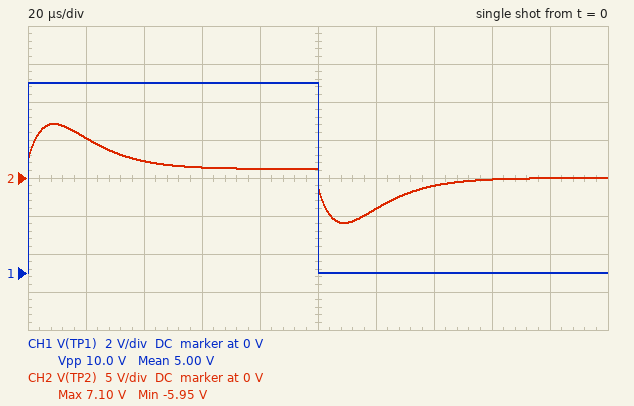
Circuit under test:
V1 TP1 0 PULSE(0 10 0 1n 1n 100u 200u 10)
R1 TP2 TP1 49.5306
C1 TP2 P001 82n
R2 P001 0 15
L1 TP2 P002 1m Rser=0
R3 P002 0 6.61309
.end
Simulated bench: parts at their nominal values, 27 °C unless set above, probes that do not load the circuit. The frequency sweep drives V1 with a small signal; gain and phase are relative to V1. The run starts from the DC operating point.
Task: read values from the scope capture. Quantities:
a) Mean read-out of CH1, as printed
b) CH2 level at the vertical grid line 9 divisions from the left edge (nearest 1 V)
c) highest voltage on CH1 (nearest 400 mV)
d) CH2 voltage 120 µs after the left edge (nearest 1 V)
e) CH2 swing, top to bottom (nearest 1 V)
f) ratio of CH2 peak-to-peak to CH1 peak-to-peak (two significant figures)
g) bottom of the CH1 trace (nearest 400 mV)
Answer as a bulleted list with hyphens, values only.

- 5.00 V
- 0 V
- 10.0 V
- -4 V
- 13 V
- 1.3
- 0 V
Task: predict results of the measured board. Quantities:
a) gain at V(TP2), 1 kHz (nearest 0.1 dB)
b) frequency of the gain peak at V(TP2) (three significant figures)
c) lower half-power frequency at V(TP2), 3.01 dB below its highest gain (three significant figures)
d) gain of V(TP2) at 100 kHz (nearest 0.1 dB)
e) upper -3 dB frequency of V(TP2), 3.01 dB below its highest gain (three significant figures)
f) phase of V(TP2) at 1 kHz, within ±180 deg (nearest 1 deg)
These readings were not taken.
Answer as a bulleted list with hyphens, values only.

- -15.8 dB
- 16.6 kHz
- 6.73 kHz
- -8.6 dB
- 42.0 kHz
- 37 deg
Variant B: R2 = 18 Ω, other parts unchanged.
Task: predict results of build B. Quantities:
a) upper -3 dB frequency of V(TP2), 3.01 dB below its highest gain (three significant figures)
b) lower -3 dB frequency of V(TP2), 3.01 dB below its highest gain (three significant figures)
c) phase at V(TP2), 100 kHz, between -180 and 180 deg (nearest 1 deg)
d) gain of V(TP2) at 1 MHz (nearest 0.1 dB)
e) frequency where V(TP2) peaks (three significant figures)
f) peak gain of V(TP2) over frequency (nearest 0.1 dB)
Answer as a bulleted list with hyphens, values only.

- 41.7 kHz
- 6.65 kHz
- -30 deg
- -11.4 dB
- 16.3 kHz
- -0.8 dB
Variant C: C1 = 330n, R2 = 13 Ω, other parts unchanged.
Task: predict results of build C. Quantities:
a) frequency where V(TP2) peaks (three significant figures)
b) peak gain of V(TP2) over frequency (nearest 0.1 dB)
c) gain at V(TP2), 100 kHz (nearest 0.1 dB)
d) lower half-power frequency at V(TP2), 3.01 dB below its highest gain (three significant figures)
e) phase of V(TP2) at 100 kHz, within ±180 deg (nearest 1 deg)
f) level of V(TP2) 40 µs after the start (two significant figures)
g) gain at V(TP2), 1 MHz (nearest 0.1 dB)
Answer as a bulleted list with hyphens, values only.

- 8.41 kHz
- -2.3 dB
- -13.1 dB
- 4.59 kHz
- -15 deg
- 3.8 V
- -13.6 dB
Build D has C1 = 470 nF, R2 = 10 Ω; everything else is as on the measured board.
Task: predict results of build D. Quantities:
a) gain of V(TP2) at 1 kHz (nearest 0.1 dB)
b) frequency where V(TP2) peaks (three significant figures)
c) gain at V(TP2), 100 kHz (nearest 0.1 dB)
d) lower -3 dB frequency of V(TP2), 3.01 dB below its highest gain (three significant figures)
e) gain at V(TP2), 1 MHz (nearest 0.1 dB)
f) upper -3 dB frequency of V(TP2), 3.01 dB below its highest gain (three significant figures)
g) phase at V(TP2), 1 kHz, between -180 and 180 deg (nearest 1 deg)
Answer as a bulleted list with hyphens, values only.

- -15.7 dB
- 7.18 kHz
- -15.0 dB
- 4.13 kHz
- -15.5 dB
- 12.7 kHz
- 36 deg
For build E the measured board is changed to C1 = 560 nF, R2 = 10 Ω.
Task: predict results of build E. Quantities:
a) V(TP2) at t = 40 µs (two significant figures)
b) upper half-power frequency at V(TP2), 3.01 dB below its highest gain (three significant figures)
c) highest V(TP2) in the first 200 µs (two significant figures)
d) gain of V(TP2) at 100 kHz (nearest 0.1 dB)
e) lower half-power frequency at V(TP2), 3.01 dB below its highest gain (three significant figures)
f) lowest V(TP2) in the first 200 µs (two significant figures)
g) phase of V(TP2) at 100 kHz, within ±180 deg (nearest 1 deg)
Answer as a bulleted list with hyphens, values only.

- 4.1 V
- 11.5 kHz
- 4.5 V
- -15.1 dB
- 3.85 kHz
- -3.7 V
- -12 deg
